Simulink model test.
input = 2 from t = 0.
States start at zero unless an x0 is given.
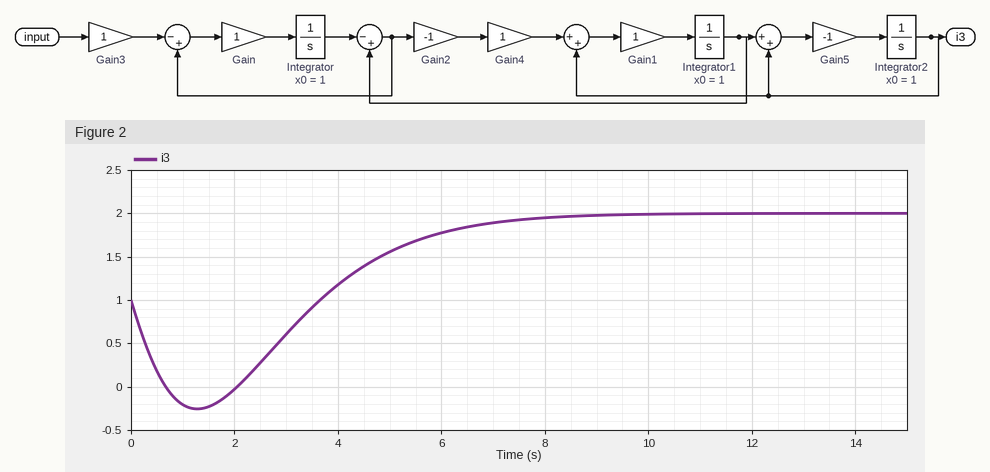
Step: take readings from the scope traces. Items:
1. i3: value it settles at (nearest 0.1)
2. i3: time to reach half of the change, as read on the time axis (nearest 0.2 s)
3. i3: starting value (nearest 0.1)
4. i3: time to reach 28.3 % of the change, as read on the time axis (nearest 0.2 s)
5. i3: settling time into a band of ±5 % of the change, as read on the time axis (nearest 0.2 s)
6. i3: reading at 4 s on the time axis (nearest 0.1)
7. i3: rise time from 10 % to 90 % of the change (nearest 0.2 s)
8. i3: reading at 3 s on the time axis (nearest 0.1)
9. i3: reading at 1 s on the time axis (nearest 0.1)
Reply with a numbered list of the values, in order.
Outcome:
1. 2.0
2. 4.8 s
3. 1.0
4. 4.2 s
5. 8.0 s
6. 1.2
7. 3.2 s
8. 0.6
9. -0.2
